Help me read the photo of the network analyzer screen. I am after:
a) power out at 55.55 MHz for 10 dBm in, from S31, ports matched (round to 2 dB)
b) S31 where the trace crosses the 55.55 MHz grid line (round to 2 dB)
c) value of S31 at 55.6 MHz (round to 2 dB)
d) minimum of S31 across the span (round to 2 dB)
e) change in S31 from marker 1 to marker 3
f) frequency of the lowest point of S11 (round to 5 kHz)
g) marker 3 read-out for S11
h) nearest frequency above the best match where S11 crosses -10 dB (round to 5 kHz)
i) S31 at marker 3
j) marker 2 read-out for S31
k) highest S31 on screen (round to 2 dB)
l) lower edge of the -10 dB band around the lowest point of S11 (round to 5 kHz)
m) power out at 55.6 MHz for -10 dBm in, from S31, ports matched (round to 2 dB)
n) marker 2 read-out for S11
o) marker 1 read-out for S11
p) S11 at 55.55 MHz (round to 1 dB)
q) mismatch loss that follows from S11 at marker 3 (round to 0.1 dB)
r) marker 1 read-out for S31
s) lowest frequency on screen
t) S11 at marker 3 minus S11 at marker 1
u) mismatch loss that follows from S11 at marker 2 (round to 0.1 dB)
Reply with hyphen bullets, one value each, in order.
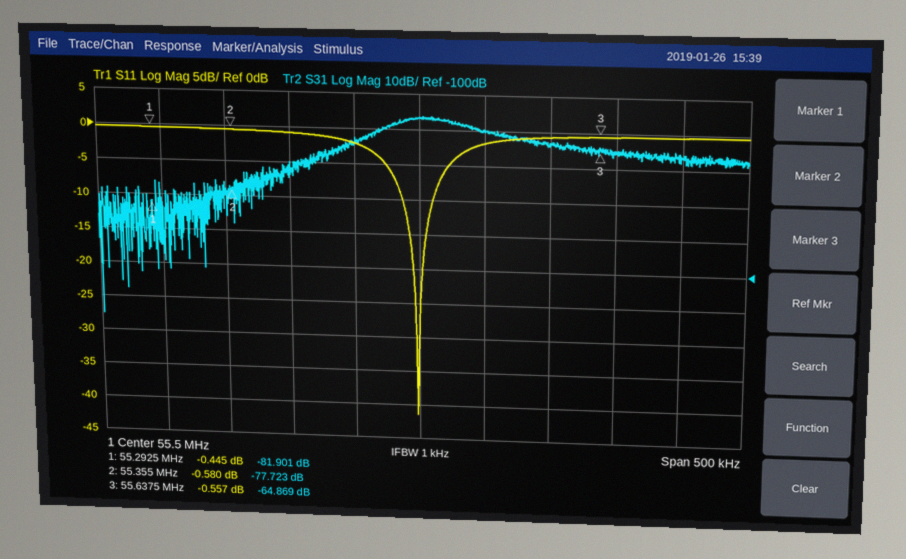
- -50 dBm
- -60 dB
- -64 dB
- -116 dB
- 17.032 dB
- 55.500 MHz
- -0.557 dB
- 55.510 MHz
- -64.869 dB
- -77.723 dB
- -56 dB
- 55.485 MHz
- -74 dBm
- -0.580 dB
- -0.445 dB
- -2 dB
- 9.2 dB
- -81.901 dB
- 55.25 MHz
- -0.112 dB
- 9.0 dB
